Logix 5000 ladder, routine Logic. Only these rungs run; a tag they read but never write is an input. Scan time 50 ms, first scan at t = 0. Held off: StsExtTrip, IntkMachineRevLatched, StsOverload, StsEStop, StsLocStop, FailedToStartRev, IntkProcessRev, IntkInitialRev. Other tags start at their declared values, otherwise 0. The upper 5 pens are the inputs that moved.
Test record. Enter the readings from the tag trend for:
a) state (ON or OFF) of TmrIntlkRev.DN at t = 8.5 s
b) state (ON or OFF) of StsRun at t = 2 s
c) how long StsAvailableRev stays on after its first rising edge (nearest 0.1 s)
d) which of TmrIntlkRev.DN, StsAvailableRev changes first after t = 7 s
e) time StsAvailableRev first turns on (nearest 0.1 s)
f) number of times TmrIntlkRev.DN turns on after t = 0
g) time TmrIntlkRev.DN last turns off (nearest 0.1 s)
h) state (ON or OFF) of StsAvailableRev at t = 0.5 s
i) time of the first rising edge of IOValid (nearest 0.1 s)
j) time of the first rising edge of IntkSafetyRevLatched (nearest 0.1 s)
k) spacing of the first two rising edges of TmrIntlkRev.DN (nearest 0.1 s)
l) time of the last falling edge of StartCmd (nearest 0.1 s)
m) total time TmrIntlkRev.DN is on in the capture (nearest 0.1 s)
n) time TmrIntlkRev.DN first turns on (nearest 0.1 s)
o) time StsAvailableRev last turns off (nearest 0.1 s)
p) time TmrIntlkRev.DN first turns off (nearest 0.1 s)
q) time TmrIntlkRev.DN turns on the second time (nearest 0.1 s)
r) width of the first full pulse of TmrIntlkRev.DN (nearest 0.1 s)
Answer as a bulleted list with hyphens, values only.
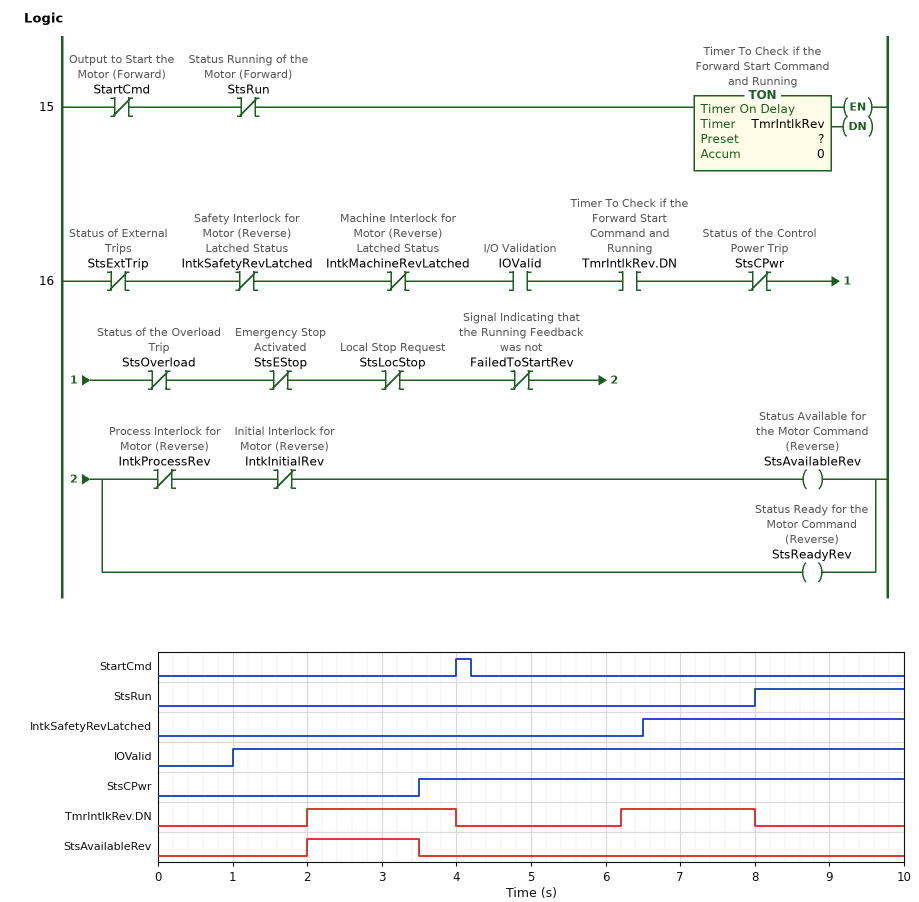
- OFF
- OFF
- 1.5 s
- TmrIntlkRev.DN
- 2.0 s
- 2
- 8.0 s
- OFF
- 1.0 s
- 6.5 s
- 4.2 s
- 4.2 s
- 3.8 s
- 2.0 s
- 3.5 s
- 4.0 s
- 6.2 s
- 2.0 s
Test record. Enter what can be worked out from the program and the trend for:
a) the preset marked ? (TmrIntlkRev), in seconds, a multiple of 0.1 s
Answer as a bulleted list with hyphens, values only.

- 2.0 s
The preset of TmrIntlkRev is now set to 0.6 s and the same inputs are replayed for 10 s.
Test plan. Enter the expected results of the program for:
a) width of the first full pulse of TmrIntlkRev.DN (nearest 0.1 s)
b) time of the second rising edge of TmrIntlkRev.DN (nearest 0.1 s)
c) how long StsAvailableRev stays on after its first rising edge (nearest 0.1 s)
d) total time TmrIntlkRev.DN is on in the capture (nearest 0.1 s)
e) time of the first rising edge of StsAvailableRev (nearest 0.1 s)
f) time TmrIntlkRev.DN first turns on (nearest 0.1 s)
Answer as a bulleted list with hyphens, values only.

- 3.4 s
- 4.8 s
- 2.5 s
- 6.6 s
- 1.0 s
- 0.6 s
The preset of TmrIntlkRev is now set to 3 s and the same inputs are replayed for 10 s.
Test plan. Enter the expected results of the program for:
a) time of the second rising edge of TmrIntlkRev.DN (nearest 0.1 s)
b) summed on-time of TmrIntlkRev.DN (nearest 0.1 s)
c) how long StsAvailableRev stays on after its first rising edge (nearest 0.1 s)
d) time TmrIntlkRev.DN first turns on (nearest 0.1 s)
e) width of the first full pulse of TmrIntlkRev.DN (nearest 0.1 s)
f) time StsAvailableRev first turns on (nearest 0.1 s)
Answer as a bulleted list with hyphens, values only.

- 7.2 s
- 1.8 s
- 0.5 s
- 3.0 s
- 1.0 s
- 3.0 s
